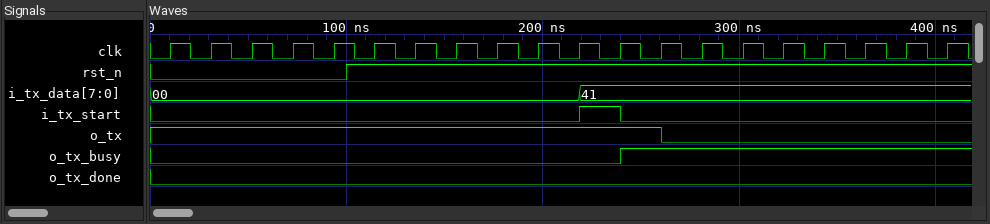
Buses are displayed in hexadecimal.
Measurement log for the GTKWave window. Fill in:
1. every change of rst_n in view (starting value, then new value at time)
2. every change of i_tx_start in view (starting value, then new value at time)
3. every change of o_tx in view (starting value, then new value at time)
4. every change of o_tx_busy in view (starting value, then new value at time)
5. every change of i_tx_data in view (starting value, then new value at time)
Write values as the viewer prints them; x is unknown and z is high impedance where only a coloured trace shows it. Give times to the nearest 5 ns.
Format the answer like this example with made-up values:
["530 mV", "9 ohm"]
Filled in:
["0, 1 at 100 ns", "0, 1 at 220 ns, 0 at 240 ns", "1, 0 at 260 ns", "0, 1 at 240 ns", "00, 41 at 220 ns"]
